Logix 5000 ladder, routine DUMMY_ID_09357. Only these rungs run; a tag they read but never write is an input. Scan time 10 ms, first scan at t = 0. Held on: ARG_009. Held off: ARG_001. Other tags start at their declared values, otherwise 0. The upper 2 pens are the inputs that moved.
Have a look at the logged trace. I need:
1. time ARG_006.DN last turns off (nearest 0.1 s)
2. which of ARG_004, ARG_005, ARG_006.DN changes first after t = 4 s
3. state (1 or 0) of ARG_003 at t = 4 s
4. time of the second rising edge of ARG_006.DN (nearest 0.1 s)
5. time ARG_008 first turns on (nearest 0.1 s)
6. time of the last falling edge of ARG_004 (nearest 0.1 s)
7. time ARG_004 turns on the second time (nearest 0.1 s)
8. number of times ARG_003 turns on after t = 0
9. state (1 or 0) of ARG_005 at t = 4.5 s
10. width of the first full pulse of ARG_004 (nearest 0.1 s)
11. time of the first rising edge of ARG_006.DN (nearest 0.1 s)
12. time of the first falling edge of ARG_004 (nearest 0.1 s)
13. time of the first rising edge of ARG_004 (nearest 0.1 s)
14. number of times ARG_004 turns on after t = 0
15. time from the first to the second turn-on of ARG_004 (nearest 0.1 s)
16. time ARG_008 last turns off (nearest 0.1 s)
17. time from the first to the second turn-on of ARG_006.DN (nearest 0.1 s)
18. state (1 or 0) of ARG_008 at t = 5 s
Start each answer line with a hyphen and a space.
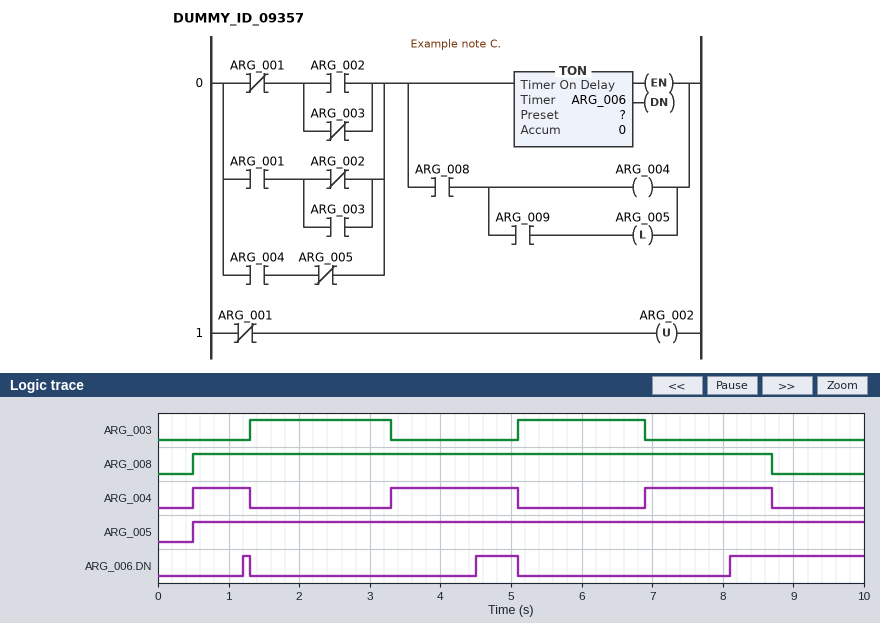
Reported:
- 5.1 s
- ARG_006.DN
- 0
- 4.5 s
- 0.5 s
- 8.7 s
- 3.3 s
- 2
- 1
- 0.8 s
- 1.2 s
- 1.3 s
- 0.5 s
- 3
- 2.8 s
- 8.7 s
- 3.3 s
- 1
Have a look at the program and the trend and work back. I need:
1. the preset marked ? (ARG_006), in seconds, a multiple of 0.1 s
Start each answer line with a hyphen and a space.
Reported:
- 1.2 s
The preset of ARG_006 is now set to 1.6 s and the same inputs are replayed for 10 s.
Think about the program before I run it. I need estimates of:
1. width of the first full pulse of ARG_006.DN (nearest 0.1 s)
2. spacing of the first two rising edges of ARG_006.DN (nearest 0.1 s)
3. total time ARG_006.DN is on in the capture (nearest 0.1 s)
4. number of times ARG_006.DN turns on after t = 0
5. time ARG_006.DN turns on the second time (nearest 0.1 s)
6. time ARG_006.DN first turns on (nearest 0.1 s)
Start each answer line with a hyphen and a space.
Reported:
- 0.2 s
- 3.6 s
- 1.7 s
- 2
- 8.5 s
- 4.9 s
